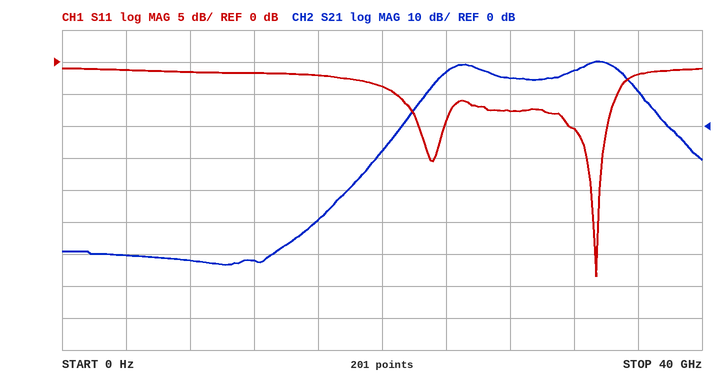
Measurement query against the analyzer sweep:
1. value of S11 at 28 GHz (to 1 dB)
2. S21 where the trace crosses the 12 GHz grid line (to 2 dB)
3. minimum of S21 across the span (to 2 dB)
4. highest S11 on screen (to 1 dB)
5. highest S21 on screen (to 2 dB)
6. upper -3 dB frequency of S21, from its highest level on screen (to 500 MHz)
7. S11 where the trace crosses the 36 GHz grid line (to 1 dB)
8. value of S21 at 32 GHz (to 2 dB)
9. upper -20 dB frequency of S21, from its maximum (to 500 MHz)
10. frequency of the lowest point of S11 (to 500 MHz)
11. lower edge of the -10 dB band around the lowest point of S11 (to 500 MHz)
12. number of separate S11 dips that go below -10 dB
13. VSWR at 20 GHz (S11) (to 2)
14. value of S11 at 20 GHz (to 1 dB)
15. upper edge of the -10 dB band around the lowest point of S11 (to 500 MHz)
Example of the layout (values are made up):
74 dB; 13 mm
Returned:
-8 dB; -42 dB; -44 dB; -1 dB; 20 dB; 35.0 GHz; -2 dB; 18 dB; 38.0 GHz; 33.5 GHz; 31.5 GHz; 2; 4; -4 dB; 34.0 GHz
